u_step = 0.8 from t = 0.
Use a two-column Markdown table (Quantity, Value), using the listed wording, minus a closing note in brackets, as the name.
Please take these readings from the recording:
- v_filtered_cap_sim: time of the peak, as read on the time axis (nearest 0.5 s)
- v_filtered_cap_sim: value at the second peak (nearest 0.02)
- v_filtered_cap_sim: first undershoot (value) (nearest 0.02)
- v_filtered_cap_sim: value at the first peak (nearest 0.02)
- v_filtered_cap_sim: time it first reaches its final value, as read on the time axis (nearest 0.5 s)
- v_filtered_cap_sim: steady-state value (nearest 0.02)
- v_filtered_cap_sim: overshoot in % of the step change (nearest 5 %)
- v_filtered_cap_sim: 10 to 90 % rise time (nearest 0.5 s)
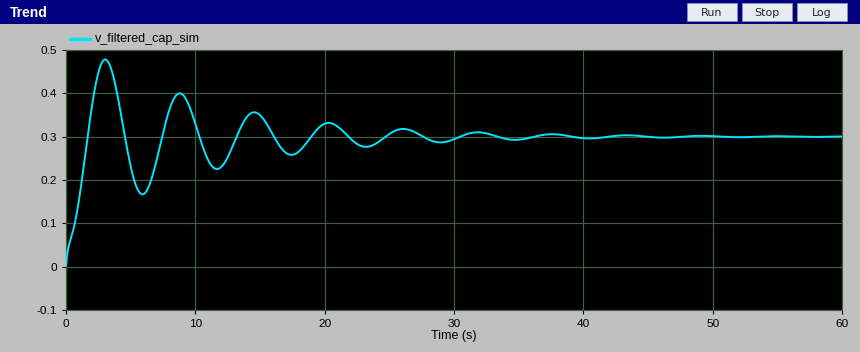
| Quantity | Value |
|---|---|
| v_filtered_cap_sim: time of the peak, as read on the time axis | 3.0 s |
| v_filtered_cap_sim: value at the second peak | 0.40 |
| v_filtered_cap_sim: first undershoot (value) | 0.16 |
| v_filtered_cap_sim: value at the first peak | 0.48 |
| v_filtered_cap_sim: time it first reaches its final value, as read on the time axis | 1.5 s |
| v_filtered_cap_sim: steady-state value | 0.30 |
| v_filtered_cap_sim: overshoot in % of the step change | 60 % |
| v_filtered_cap_sim: 10 to 90 % rise time | 1.5 s |
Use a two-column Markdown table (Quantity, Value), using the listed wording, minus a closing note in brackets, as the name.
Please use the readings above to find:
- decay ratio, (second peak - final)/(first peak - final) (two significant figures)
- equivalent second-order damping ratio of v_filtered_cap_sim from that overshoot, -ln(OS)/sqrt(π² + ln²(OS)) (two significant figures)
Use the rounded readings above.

| Quantity | Value |
|---|---|
| decay ratio, (second peak - final)/(first peak - final) | 0.56 |
| equivalent second-order damping ratio of v_filtered_cap_sim from that overshoot, -ln(OS)/sqrt(π² + ln²(OS)) | 0.16 |
